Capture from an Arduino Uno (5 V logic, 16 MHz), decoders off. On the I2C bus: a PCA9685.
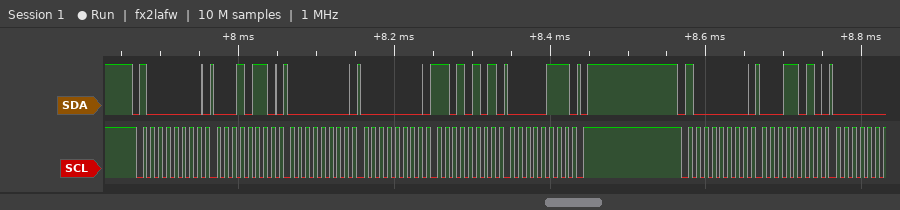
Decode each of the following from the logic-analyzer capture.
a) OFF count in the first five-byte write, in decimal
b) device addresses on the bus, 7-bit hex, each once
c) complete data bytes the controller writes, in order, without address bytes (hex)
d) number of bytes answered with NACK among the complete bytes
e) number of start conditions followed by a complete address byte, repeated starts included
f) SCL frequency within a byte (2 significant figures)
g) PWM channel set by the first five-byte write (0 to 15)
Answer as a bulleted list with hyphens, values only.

- 2005
- 0x40
- 16 00 00 D5 07 1A
- 0
- 2
- 100 kHz
- 4
